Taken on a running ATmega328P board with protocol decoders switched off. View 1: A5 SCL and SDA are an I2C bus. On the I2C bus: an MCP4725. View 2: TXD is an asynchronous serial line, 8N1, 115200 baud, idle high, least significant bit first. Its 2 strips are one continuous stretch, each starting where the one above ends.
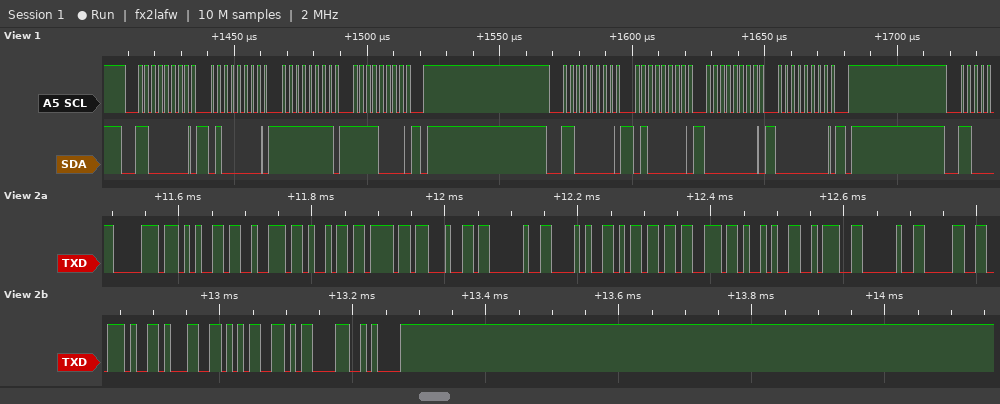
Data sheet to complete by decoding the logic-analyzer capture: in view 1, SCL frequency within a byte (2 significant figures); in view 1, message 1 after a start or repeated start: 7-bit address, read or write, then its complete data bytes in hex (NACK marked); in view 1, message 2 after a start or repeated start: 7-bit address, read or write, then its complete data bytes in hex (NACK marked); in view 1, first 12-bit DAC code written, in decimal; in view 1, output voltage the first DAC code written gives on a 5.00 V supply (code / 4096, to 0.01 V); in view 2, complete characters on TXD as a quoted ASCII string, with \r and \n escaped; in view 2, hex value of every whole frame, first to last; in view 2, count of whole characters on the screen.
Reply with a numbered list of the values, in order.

1. 400 kHz
2. 0x60 write: 40 FF F0
3. 0x60 write: 40 00 00
4. 4095
5. 5.00 V
6. "period (ms): 0.15\r\n"
7. 0x70 0x65 0x72 0x69 0x6F 0x64 0x20 0x28 0x6D 0x73 0x29 0x3A 0x20 0x30 0x2E 0x31 0x35 0x0D 0x0A
8. 19
